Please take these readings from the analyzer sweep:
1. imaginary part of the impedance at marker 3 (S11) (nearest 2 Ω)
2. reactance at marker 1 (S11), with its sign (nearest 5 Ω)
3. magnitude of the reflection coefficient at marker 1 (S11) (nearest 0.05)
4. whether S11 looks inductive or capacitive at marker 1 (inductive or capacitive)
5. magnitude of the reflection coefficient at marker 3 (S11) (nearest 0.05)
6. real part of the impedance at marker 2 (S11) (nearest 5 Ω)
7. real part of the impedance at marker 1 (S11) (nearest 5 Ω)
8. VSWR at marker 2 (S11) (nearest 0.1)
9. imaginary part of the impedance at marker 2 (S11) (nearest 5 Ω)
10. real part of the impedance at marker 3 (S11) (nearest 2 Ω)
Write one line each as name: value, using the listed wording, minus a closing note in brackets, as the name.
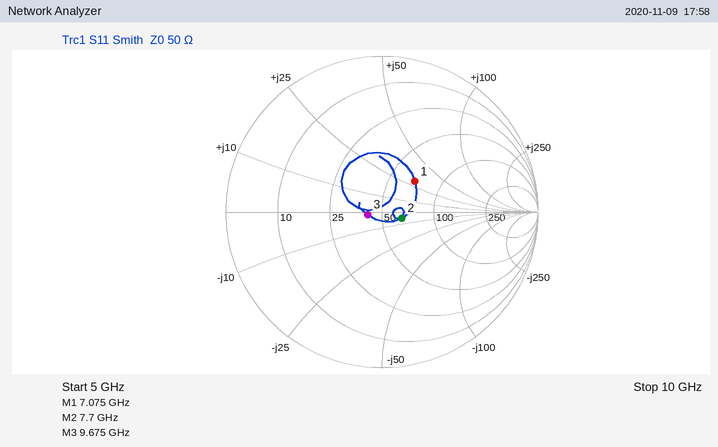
imaginary part of the impedance at marker 3 (S11): -2 Ω
reactance at marker 1 (S11), with its sign: +30 Ω
magnitude of the reflection coefficient at marker 1 (S11): 0.30
whether S11 looks inductive or capacitive at marker 1: inductive
magnitude of the reflection coefficient at marker 3 (S11): 0.10
real part of the impedance at marker 2 (S11): 65 Ω
real part of the impedance at marker 1 (S11): 70 Ω
VSWR at marker 2 (S11): 1.3
imaginary part of the impedance at marker 2 (S11): -5 Ω
real part of the impedance at marker 3 (S11): 42 Ω
